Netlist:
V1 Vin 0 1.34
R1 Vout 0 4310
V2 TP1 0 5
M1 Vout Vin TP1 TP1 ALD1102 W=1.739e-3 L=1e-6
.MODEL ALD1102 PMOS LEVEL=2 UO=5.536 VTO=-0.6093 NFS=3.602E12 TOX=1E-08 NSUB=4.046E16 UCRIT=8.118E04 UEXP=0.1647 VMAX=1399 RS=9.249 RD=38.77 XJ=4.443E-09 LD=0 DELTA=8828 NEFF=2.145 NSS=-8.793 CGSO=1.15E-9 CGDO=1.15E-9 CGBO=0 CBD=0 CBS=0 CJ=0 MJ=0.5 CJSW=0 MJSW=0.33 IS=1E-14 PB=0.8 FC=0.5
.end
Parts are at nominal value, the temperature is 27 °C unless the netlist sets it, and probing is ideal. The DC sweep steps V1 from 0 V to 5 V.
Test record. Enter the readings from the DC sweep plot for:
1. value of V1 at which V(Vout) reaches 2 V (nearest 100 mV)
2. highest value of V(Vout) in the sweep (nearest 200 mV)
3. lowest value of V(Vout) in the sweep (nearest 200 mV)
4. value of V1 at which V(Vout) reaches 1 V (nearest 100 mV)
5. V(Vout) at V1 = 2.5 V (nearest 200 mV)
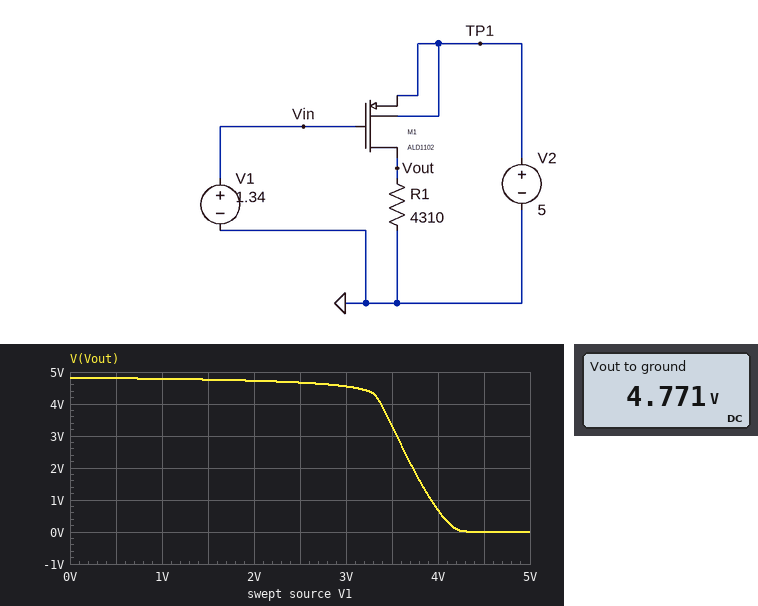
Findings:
3.7 V
4.8 V
0 V
3.9 V
4.6 V
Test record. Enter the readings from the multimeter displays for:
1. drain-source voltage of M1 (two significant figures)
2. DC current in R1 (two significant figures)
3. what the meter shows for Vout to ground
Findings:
-230 mV
1.1 mA
4.771 V
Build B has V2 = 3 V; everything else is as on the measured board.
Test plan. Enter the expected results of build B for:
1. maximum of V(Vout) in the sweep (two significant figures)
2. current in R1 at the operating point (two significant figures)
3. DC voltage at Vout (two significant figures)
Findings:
2.8 V
620 µA
2.7 V
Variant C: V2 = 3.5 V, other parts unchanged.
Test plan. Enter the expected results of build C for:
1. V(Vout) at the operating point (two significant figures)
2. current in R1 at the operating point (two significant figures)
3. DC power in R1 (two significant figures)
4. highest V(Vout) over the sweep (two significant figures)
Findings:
3.2 V
750 µA
2.4 mW
3.3 V
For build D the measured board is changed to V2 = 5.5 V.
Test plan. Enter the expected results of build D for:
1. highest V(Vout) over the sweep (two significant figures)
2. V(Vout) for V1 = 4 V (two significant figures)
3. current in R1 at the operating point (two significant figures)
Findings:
5.3 V
3.4 V
1.2 mA
